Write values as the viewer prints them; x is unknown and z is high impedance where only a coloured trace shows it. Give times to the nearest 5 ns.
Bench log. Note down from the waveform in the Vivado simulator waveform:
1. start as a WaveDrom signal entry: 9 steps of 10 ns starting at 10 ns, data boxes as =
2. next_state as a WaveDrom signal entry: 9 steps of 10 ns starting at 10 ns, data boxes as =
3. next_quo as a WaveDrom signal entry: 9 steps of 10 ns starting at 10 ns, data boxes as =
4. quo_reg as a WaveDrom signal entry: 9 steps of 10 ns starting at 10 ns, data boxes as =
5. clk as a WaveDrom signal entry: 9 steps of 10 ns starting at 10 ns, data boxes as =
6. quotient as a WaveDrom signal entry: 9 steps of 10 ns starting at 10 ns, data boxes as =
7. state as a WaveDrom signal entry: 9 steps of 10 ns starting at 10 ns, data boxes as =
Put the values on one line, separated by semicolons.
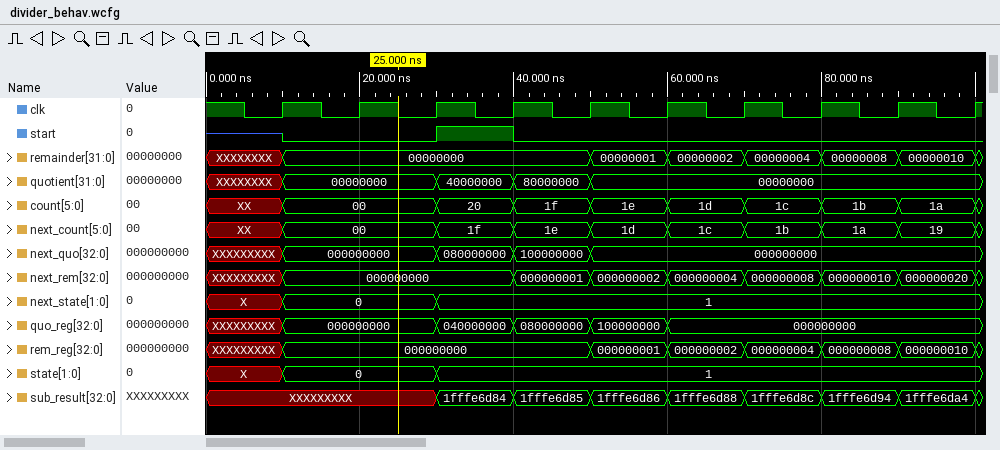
{name: 'start', wave: '0.10.....'}; {name: 'next_state', wave: '=.=......', data: '0 1'}; {name: 'next_quo', wave: '=.===....', data: '000000000 080000000 100000000 000000000'}; {name: 'quo_reg', wave: '=.====...', data: '000000000 040000000 080000000 100000000 000000000'}; {name: 'clk', wave: 'p........'}; {name: 'quotient', wave: '=.===....', data: '00000000 40000000 80000000 00000000'}; {name: 'state', wave: '=.=......', data: '0 1'}
